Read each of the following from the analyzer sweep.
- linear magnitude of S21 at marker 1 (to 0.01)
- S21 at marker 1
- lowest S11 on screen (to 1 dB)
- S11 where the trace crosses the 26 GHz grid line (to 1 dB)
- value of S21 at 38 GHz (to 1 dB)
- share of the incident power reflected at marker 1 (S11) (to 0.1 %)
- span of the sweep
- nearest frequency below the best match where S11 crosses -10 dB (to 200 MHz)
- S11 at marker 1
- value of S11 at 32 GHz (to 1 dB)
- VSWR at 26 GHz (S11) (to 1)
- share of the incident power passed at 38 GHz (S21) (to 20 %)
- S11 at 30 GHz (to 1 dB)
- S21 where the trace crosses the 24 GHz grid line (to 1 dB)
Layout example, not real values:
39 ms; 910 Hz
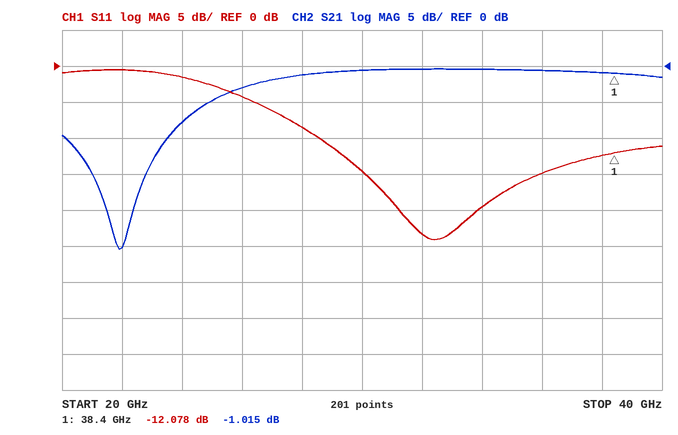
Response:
0.89; -1.015 dB; -24 dB; -4 dB; -1 dB; 6.2 %; 20 GHz; 28.6 GHz; -12.078 dB; -23 dB; 4; 80 %; -15 dB; -8 dB
